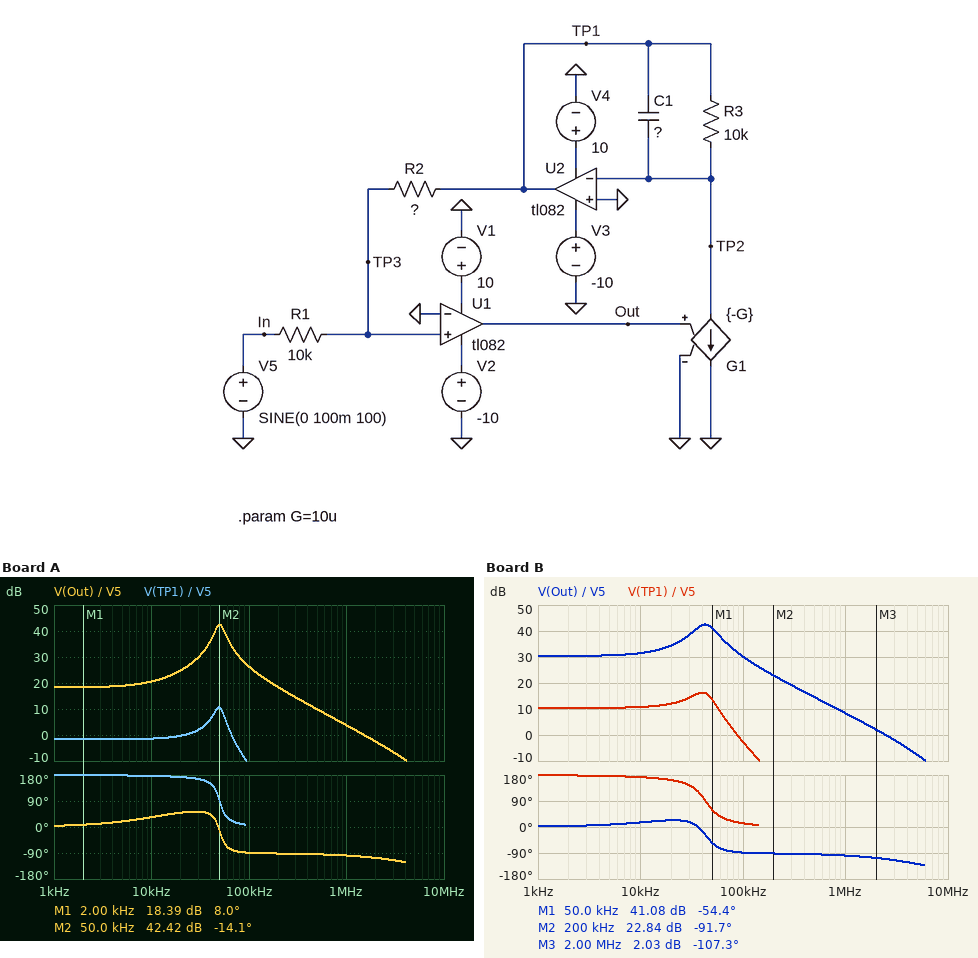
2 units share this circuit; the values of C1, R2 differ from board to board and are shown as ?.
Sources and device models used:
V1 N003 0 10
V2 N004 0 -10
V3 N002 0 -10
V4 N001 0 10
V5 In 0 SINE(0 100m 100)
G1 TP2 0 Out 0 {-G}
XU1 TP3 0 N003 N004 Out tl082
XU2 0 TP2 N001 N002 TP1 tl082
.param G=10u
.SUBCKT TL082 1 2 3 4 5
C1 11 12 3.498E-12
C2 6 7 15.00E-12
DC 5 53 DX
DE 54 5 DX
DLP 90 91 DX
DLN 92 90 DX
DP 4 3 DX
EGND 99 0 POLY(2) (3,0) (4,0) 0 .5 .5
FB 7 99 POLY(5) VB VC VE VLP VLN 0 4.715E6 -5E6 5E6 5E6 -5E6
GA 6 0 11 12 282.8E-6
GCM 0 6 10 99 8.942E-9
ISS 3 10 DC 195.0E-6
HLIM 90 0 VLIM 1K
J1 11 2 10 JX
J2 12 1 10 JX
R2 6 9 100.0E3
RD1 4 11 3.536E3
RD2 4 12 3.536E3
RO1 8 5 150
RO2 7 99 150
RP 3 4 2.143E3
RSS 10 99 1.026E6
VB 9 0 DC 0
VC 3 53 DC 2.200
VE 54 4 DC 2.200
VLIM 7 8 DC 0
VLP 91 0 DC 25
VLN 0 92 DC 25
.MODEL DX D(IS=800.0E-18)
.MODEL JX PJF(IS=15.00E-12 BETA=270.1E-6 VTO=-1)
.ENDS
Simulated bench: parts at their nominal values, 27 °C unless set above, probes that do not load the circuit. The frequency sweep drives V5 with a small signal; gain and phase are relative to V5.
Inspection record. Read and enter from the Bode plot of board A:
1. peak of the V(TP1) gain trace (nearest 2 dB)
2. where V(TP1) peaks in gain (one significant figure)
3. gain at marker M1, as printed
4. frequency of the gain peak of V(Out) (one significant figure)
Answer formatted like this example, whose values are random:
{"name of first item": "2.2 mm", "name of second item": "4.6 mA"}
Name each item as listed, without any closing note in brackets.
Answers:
{"peak of the V(TP1) gain trace": "10 dB", "where V(TP1) peaks in gain": "50 kHz", "gain at marker M1, as printed": "18.39 dB", "frequency of the gain peak of V(Out)": "50 kHz"}
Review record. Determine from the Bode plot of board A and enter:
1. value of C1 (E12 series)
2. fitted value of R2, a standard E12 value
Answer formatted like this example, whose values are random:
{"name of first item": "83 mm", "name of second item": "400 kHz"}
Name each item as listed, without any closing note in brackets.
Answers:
{"value of C1": "1.2 nF", "fitted value of R2, a standard E12 value": "8.2 kΩ"}
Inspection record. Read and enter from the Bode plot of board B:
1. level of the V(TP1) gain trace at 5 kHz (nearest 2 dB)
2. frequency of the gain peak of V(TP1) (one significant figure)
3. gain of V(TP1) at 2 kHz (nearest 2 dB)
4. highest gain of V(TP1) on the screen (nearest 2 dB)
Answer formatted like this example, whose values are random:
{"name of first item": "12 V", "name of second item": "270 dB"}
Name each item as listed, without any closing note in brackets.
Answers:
{"level of the V(TP1) gain trace at 5 kHz": "10 dB", "frequency of the gain peak of V(TP1)": "40 kHz", "gain of V(TP1) at 2 kHz": "10 dB", "highest gain of V(TP1) on the screen": "16 dB"}
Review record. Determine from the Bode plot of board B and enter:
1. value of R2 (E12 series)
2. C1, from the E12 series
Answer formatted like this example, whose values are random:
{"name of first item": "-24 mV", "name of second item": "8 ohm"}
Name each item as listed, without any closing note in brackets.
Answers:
{"value of R2": "33 kΩ", "C1, from the E12 series": "680 pF"}
